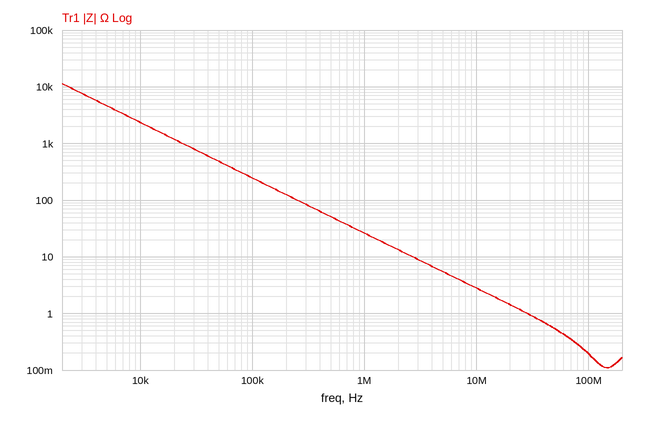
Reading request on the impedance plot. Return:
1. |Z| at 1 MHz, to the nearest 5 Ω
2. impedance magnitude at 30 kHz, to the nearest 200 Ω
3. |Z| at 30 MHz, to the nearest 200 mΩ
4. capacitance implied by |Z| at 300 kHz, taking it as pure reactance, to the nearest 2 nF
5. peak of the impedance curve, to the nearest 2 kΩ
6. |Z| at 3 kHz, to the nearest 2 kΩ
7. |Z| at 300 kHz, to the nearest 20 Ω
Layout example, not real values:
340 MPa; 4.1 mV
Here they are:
25 Ω; 800 Ω; 1.0 Ω; 6 nF; 12 kΩ; 8 kΩ; 80 Ω
